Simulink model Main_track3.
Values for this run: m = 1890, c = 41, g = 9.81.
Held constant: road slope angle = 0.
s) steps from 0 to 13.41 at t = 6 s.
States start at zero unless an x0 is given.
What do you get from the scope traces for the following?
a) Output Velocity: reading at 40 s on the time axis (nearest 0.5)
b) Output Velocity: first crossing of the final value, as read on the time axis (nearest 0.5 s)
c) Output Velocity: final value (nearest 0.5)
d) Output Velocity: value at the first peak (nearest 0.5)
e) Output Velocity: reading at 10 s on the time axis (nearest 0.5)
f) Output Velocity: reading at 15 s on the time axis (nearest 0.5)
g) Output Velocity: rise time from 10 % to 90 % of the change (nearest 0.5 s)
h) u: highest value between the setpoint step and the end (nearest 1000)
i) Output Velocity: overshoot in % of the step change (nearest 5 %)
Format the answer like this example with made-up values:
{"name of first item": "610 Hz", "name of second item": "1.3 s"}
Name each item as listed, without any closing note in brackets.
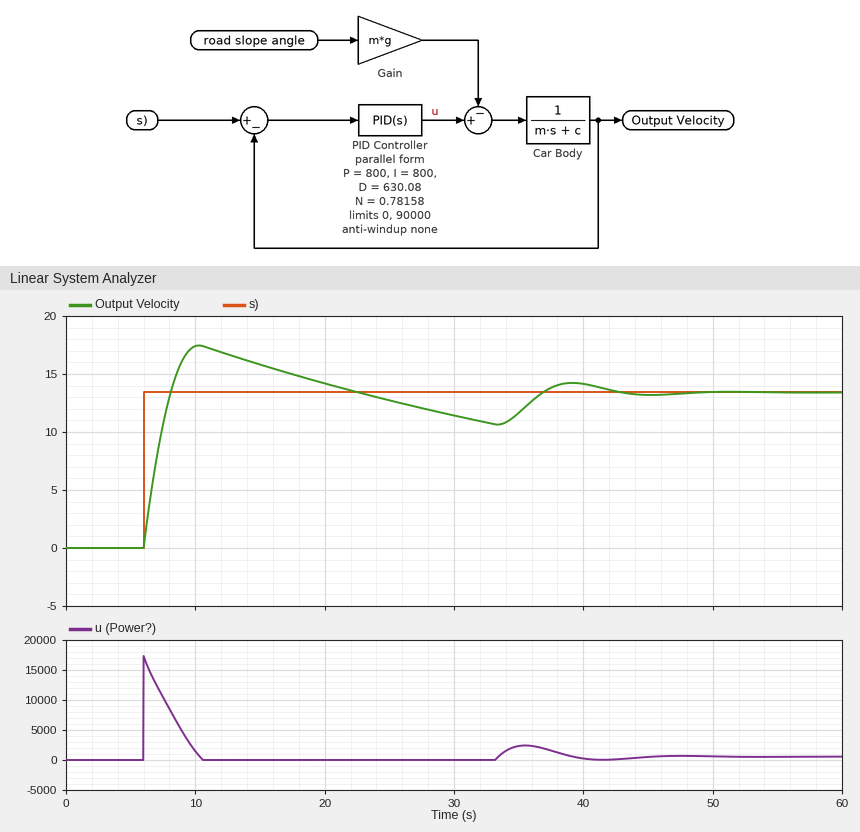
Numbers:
{"Output Velocity: reading at 40 s on the time axis": "14.0", "Output Velocity: first crossing of the final value, as read on the time axis": "8.0 s", "Output Velocity: final value": "13.5", "Output Velocity: value at the first peak": "17.5", "Output Velocity: reading at 10 s on the time axis": "17.5", "Output Velocity: reading at 15 s on the time axis": "16.0", "Output Velocity: rise time from 10 % to 90 % of the change": "1.5 s", "u: highest value between the setpoint step and the end": "17000", "Output Velocity: overshoot in % of the step change": "30 %"}
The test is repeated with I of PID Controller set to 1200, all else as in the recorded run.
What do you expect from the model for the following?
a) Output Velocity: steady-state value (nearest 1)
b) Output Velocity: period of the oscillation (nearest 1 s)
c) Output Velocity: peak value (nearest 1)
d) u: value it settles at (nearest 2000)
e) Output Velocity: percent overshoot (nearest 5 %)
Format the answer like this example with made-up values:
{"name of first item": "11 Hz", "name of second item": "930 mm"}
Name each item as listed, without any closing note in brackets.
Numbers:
{"Output Velocity: steady-state value": "13", "Output Velocity: period of the oscillation": "32 s", "Output Velocity: peak value": "18", "u: value it settles at": "0", "Output Velocity: percent overshoot": "35 %"}
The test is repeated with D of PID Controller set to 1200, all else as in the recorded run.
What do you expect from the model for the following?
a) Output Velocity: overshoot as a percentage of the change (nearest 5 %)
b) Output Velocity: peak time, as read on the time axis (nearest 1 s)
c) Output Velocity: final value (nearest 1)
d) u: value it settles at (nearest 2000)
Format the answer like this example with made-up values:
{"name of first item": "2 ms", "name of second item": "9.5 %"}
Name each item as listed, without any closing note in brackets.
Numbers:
{"Output Velocity: overshoot as a percentage of the change": "25 %", "Output Velocity: peak time, as read on the time axis": "11 s", "Output Velocity: final value": "13", "u: value it settles at": "0"}
